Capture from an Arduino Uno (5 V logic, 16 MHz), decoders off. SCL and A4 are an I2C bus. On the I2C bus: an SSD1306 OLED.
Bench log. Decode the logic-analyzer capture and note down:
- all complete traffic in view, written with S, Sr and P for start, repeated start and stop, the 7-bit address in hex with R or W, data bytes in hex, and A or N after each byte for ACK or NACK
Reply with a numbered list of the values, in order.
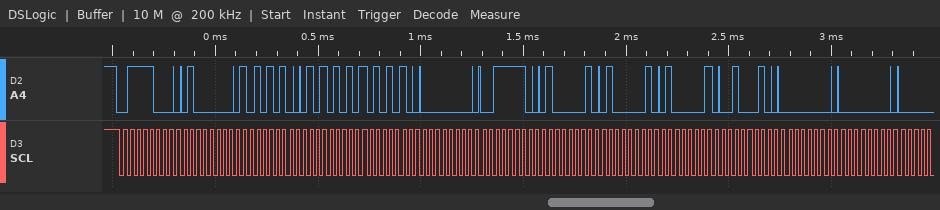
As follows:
1. S 3CW A 40 A AA A 55 A AA A 00 A 3E A 41 A 41 A 41 A 22 A 00 A 00 A
